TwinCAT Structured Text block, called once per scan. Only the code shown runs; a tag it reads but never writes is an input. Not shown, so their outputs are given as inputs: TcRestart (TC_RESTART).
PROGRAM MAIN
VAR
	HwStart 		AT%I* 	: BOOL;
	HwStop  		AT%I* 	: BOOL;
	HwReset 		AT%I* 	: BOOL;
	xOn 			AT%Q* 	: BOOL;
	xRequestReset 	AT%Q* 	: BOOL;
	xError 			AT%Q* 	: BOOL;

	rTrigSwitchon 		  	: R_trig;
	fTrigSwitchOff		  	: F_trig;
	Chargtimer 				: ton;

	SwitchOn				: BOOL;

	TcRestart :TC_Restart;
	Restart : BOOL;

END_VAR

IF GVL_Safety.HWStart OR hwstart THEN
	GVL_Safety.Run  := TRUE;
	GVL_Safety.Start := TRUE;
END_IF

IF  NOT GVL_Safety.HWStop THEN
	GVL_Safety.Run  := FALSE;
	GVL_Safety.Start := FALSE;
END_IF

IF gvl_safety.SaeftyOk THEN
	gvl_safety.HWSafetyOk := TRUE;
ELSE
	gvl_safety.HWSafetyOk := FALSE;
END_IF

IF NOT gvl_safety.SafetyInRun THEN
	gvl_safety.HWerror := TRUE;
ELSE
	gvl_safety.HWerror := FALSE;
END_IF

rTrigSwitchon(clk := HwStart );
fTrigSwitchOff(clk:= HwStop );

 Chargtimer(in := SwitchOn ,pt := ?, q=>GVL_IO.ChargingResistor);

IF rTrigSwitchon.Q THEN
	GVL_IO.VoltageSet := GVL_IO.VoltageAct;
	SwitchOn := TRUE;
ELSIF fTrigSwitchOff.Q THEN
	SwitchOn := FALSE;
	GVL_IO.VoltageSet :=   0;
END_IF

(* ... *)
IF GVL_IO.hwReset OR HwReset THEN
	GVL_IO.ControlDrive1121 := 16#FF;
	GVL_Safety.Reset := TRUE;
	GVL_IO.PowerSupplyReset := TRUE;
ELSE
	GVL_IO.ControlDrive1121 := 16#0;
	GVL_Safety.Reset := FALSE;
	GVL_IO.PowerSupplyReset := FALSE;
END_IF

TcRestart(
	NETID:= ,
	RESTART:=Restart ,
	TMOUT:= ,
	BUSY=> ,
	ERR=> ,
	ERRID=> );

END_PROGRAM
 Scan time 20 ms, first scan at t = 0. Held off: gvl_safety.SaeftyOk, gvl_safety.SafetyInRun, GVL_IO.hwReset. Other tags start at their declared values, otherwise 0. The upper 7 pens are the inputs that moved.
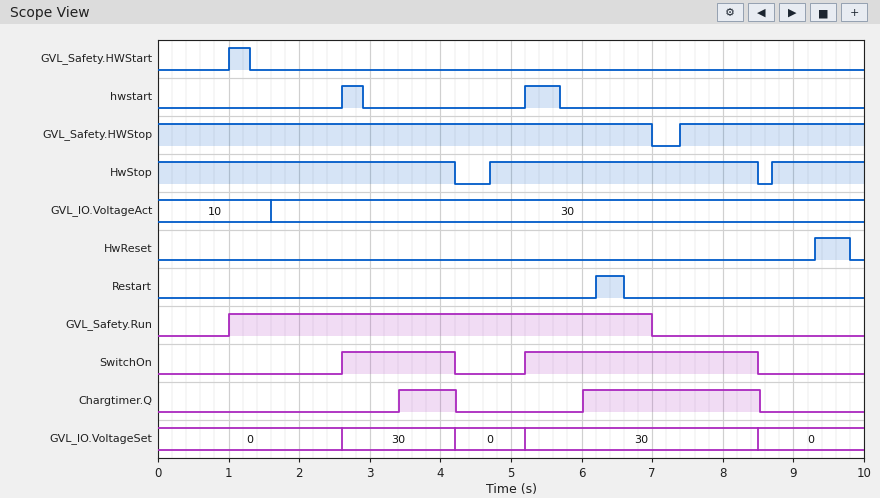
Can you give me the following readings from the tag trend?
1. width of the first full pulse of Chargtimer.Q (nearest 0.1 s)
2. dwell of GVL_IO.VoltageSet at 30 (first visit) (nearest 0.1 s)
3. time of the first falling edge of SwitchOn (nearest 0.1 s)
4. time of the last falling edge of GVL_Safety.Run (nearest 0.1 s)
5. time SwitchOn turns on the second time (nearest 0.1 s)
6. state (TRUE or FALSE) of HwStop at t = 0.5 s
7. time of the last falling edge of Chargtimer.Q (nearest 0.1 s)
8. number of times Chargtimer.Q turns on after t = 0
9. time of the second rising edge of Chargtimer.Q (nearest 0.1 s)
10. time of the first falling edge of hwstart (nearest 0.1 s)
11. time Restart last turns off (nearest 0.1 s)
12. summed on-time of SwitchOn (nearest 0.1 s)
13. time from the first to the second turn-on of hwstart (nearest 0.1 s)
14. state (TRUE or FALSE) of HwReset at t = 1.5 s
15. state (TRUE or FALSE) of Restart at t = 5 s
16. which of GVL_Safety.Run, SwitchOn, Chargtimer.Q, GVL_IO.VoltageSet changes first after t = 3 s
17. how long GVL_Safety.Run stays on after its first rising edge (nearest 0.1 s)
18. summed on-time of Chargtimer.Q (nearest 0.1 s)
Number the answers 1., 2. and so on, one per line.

1. 0.8 s
2. 1.6 s
3. 4.2 s
4. 7.0 s
5. 5.2 s
6. TRUE
7. 8.5 s
8. 2
9. 6.0 s
10. 2.9 s
11. 6.6 s
12. 4.9 s
13. 2.6 s
14. FALSE
15. FALSE
16. Chargtimer.Q
17. 6.0 s
18. 3.3 s
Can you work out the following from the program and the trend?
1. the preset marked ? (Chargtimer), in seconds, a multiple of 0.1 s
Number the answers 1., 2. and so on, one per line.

1. 0.8 s
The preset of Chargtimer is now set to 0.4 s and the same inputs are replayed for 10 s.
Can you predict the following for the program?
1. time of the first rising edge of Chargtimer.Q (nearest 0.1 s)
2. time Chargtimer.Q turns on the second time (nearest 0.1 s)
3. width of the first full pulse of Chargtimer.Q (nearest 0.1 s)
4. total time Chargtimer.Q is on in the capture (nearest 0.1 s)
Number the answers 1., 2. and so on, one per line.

1. 3.0 s
2. 5.6 s
3. 1.2 s
4. 4.1 s
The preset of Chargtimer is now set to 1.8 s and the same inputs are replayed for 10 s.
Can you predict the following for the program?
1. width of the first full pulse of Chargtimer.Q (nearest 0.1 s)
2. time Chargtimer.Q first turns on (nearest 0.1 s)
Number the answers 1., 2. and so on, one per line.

1. 1.5 s
2. 7.0 s
